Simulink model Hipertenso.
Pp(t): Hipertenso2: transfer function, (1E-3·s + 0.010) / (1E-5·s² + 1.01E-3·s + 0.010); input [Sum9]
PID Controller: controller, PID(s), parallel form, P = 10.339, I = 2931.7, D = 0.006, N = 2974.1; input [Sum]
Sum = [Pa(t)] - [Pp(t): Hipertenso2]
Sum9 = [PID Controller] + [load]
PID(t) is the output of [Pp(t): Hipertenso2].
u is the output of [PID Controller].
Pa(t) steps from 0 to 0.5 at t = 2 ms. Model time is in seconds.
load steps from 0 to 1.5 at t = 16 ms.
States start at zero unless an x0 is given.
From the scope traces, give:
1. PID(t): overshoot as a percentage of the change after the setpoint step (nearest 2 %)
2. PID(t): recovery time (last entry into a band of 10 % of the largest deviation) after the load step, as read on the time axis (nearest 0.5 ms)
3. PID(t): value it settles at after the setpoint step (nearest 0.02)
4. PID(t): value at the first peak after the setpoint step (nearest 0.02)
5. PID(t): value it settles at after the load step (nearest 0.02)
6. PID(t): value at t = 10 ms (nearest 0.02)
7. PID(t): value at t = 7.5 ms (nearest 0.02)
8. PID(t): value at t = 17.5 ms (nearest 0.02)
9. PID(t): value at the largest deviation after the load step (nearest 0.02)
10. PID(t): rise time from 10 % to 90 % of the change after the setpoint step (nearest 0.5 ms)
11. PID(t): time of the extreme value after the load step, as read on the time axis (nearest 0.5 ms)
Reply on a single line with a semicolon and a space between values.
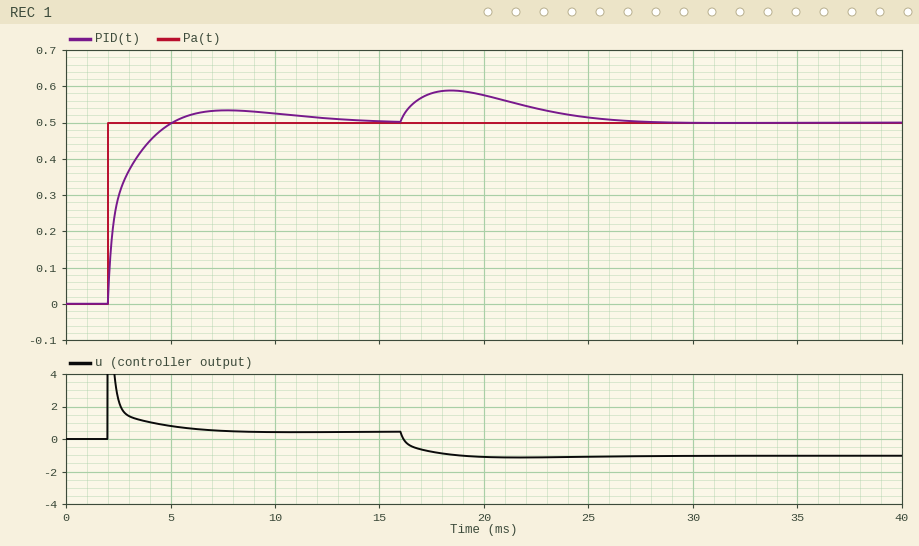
6 %; 26.0 ms; 0.50; 0.54; 0.50; 0.52; 0.54; 0.58; 0.58; 2.0 ms; 18.5 ms
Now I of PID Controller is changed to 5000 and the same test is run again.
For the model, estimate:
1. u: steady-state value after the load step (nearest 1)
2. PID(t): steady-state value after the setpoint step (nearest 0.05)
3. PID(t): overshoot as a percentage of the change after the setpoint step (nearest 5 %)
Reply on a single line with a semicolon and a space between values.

-1; 0.50; 10 %
